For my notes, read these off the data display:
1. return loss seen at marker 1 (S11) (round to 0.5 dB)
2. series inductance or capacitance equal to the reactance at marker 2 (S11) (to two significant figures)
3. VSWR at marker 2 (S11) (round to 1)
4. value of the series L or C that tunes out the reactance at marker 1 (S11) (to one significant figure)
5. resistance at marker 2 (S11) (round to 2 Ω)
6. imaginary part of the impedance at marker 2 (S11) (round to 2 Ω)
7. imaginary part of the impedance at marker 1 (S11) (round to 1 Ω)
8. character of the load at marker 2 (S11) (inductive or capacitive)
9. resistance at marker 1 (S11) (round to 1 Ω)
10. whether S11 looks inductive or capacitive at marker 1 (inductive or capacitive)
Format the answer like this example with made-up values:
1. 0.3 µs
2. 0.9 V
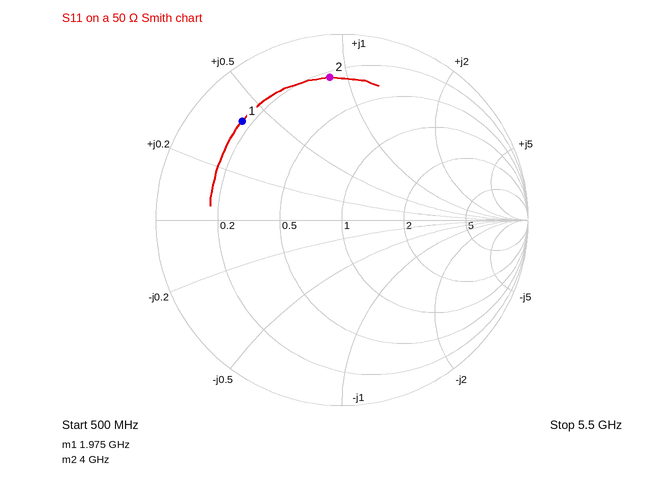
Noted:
1. 2.5 dB
2. 1.8 nH
3. 8
4. 4 pF
5. 12 Ω
6. +44 Ω
7. +20 Ω
8. inductive
9. 8 Ω
10. inductive
